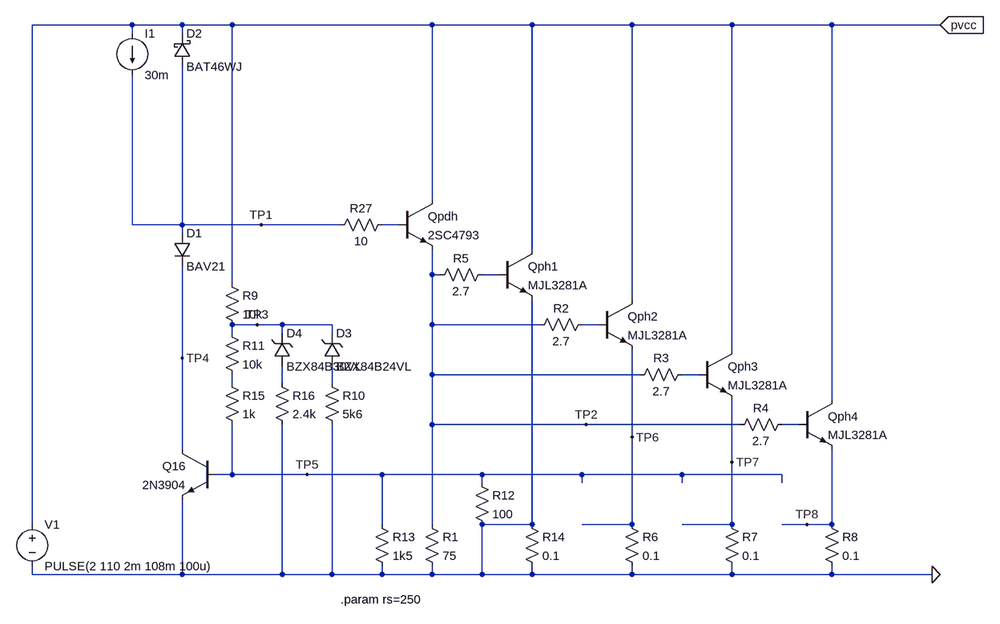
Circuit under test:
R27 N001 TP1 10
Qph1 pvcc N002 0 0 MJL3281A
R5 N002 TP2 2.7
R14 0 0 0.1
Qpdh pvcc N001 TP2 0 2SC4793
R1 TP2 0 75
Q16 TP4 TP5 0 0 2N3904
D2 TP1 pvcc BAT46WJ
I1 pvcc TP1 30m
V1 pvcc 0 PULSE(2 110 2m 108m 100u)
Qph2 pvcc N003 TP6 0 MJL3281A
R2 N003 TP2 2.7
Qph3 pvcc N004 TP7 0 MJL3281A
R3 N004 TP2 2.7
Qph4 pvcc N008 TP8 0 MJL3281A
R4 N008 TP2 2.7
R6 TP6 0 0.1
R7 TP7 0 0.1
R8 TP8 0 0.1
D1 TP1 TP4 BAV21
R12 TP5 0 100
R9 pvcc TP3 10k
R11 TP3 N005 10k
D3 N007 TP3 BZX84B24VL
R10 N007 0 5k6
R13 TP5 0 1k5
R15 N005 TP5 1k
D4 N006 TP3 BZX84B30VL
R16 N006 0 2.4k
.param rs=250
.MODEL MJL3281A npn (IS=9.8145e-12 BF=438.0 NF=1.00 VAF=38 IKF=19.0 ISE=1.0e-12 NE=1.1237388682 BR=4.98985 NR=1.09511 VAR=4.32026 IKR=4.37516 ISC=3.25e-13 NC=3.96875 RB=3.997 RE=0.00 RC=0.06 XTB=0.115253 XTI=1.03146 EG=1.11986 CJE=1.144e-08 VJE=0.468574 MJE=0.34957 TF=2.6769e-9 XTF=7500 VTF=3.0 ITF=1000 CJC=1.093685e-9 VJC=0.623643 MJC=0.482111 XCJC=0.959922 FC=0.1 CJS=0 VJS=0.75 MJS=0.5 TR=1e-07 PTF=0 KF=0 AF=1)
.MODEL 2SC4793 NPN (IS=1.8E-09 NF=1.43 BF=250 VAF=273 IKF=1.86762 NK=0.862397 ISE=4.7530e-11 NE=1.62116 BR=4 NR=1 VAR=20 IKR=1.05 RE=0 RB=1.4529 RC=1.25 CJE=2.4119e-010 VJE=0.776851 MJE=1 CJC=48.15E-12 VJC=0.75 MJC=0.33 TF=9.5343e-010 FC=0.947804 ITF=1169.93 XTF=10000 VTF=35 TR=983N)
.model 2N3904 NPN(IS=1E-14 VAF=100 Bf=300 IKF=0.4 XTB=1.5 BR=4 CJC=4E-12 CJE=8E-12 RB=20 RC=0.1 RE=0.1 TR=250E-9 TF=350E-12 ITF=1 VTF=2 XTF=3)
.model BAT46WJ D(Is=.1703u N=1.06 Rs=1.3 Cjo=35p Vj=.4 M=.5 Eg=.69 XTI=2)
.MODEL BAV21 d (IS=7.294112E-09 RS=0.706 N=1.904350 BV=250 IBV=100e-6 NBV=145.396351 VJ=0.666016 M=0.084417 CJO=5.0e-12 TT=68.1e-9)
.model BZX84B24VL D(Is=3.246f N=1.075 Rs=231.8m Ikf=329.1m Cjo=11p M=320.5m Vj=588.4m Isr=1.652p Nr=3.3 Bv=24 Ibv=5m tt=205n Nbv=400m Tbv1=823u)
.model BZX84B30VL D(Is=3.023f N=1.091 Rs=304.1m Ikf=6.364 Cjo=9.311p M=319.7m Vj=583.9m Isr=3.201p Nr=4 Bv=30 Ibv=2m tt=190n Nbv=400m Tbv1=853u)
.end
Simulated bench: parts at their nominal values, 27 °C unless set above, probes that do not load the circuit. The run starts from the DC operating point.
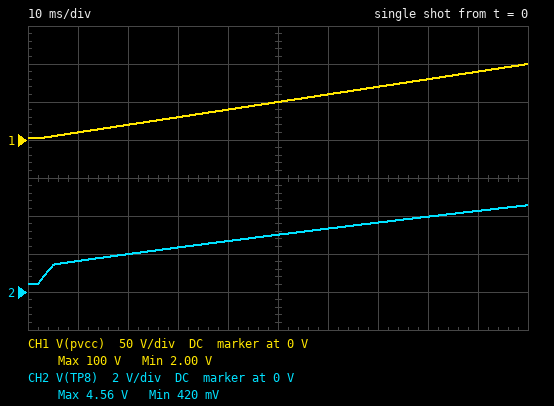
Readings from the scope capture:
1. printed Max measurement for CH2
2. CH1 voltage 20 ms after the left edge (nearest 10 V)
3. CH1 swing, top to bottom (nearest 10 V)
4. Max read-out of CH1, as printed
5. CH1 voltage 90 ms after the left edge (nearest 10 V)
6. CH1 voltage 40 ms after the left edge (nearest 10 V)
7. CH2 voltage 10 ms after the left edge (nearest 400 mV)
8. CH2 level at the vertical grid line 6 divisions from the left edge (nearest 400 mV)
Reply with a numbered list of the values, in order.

1. 4.56 V
2. 20 V
3. 100 V
4. 100 V
5. 90 V
6. 40 V
7. 1.6 V
8. 3.2 V
